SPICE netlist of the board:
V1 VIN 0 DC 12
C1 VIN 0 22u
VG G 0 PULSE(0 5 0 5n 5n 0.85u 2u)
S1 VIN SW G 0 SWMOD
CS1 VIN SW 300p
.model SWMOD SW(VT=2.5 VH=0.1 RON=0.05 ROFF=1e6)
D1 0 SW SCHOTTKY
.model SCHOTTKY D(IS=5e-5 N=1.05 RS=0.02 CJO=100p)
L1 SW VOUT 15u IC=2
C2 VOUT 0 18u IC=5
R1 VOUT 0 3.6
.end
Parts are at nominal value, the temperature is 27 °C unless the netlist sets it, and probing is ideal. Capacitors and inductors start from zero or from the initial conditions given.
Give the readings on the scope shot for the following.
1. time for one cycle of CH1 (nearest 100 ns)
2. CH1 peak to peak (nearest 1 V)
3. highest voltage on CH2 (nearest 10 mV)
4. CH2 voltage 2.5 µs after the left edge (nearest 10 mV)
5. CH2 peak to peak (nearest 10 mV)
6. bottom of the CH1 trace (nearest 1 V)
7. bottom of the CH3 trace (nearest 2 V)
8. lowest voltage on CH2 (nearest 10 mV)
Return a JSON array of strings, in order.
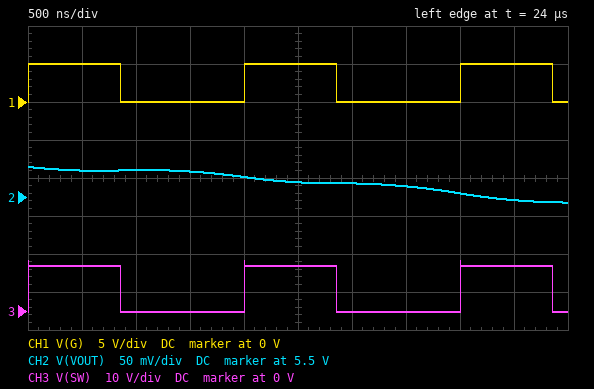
["2.0 µs", "5 V", "5.54 V", "5.52 V", "50 mV", "0 V", "0 V", "5.49 V"]
